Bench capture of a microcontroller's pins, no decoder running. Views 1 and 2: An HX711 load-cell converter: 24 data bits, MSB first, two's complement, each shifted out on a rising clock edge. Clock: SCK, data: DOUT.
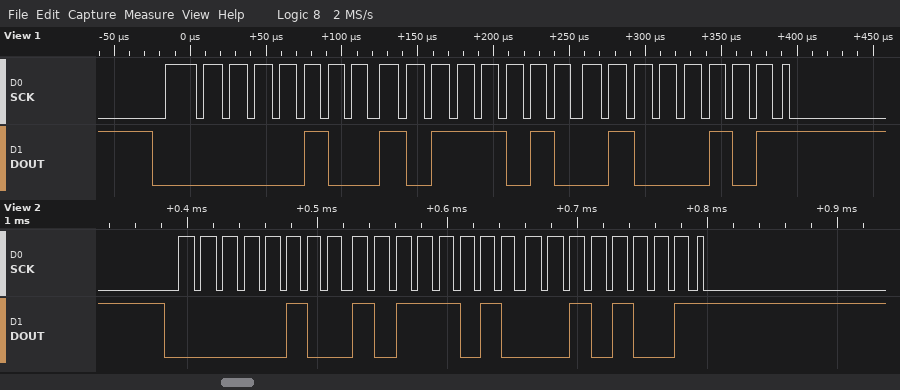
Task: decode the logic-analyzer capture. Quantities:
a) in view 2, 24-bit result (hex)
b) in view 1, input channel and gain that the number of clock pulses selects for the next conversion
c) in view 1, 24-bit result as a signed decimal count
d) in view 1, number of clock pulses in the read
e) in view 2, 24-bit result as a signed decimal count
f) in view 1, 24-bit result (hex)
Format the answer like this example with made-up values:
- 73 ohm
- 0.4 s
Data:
- 0x04BA29
- channel A, gain 128
- 309829
- 25
- 309801
- 0x04BA45
